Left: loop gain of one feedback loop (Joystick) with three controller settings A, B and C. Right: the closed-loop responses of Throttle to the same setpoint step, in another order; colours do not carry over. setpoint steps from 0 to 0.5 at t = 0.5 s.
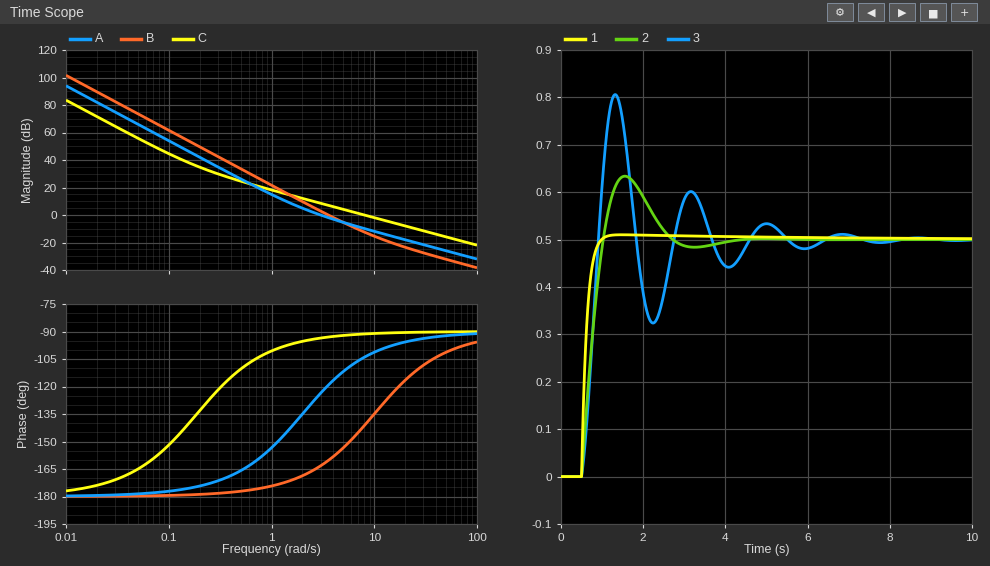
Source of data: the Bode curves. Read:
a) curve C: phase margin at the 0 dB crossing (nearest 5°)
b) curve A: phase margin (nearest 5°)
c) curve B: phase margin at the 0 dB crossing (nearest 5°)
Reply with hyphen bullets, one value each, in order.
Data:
- 90°
- 55°
- 20°
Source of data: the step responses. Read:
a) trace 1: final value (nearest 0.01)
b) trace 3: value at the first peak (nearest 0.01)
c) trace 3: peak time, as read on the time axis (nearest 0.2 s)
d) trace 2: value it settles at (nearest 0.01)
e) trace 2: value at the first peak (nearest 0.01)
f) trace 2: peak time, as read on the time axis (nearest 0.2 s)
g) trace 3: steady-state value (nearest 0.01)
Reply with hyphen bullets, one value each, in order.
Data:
- 0.50
- 0.81
- 1.4 s
- 0.50
- 0.63
- 1.6 s
- 0.50
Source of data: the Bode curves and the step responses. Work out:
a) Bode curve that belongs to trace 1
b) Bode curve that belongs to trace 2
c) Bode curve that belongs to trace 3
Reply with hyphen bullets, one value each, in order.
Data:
- C
- A
- B
